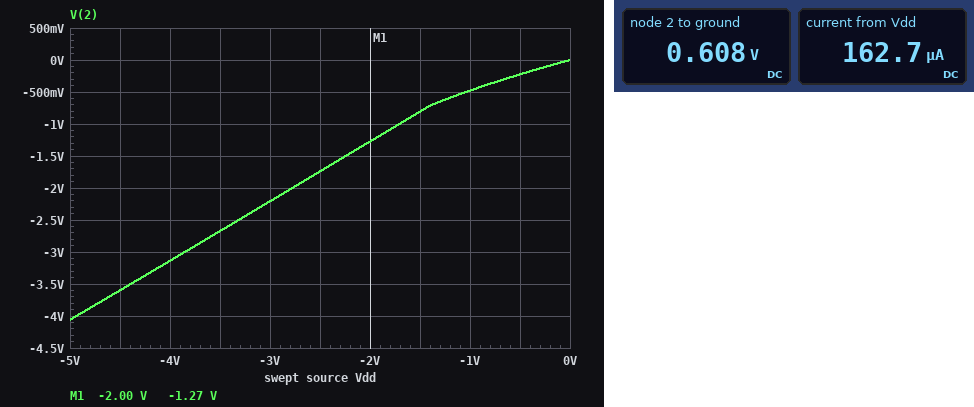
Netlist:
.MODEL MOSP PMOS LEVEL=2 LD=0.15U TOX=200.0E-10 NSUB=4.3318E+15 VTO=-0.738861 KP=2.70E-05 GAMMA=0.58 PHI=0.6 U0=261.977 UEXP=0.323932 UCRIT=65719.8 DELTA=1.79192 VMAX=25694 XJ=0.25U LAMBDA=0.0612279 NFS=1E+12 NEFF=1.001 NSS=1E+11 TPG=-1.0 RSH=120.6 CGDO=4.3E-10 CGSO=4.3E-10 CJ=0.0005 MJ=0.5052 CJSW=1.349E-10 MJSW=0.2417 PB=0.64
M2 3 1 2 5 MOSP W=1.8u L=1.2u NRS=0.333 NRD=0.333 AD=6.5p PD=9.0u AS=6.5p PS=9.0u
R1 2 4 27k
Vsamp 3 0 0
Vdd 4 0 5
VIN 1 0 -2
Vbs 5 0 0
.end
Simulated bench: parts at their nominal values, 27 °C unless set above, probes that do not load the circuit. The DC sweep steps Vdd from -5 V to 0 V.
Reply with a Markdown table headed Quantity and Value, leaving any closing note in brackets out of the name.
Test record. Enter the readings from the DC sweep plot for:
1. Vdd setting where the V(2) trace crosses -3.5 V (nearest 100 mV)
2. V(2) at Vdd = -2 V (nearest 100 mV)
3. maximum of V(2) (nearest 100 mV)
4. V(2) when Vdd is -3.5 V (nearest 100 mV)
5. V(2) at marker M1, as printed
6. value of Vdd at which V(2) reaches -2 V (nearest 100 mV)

| Quantity | Value |
|---|---|
| Vdd setting where the V(2) trace crosses -3.5 V | -4.4 V |
| V(2) at Vdd = -2 V | -1.3 V |
| maximum of V(2) | 0 V |
| V(2) when Vdd is -3.5 V | -2.7 V |
| V(2) at marker M1, as printed | -1.27 V |
| value of Vdd at which V(2) reaches -2 V | -2.8 V |
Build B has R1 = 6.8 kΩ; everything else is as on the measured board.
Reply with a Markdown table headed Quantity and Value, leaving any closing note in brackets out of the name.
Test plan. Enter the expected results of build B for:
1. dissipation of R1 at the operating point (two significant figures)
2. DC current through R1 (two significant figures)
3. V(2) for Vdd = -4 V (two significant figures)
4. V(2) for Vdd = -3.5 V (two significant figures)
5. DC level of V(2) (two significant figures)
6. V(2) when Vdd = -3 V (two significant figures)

| Quantity | Value |
|---|---|
| dissipation of R1 at the operating point | 2.8 mW |
| DC current through R1 | 640 µA |
| V(2) for Vdd = -4 V | -3.8 V |
| V(2) for Vdd = -3.5 V | -3.3 V |
| DC level of V(2) | 670 mV |
| V(2) when Vdd = -3 V | -2.8 V |
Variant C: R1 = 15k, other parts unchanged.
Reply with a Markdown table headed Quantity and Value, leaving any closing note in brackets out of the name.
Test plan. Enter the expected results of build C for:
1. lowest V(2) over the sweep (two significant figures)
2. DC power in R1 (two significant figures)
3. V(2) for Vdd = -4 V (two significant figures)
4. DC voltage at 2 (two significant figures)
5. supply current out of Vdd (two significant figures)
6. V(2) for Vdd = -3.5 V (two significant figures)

| Quantity | Value |
|---|---|
| lowest V(2) over the sweep | -4.5 V |
| DC power in R1 | 1.3 mW |
| V(2) for Vdd = -4 V | -3.5 V |
| DC voltage at 2 | 630 mV |
| supply current out of Vdd | 290 µA |
| V(2) for Vdd = -3.5 V | -3.0 V |
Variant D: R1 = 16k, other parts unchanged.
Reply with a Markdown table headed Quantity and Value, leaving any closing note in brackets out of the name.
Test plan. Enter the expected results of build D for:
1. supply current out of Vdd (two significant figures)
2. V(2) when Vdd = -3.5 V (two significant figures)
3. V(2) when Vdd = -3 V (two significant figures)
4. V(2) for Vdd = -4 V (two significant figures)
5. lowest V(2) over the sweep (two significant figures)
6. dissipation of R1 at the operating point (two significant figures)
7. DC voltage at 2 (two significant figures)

| Quantity | Value |
|---|---|
| supply current out of Vdd | 270 µA |
| V(2) when Vdd = -3.5 V | -3.0 V |
| V(2) when Vdd = -3 V | -2.5 V |
| V(2) for Vdd = -4 V | -3.5 V |
| lowest V(2) over the sweep | -4.4 V |
| dissipation of R1 at the operating point | 1.2 mW |
| DC voltage at 2 | 630 mV |
